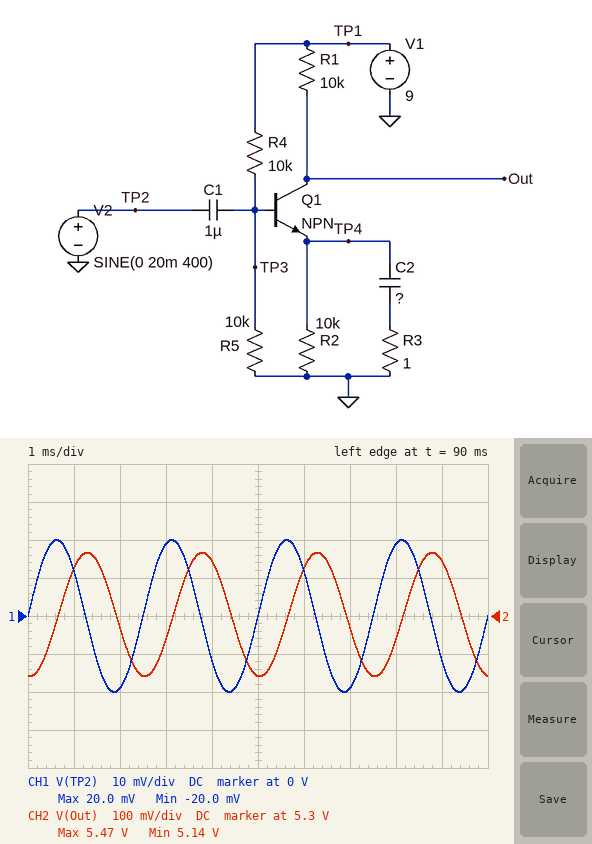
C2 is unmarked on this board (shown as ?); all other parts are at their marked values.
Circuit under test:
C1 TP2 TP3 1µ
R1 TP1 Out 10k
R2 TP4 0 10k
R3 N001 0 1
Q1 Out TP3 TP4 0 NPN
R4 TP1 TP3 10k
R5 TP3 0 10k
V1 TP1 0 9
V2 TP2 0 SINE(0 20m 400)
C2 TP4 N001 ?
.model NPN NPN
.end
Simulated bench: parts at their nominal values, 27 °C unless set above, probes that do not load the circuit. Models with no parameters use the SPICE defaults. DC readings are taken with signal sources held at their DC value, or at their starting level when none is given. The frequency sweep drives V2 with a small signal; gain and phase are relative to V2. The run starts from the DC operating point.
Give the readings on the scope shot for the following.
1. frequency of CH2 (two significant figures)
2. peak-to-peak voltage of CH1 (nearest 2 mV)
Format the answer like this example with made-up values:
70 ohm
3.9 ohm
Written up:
400 Hz
40 mV
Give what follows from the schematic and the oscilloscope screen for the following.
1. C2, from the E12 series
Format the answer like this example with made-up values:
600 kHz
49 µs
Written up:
330 nF
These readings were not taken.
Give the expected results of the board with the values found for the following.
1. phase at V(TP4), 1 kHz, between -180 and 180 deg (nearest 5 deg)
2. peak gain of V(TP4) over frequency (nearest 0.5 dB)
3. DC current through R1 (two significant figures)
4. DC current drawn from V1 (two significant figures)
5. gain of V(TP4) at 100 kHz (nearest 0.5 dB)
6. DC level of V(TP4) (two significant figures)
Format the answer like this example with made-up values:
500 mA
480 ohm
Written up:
-5 deg
0 dB
370 µA
820 µA
-23.0 dB
3.7 V
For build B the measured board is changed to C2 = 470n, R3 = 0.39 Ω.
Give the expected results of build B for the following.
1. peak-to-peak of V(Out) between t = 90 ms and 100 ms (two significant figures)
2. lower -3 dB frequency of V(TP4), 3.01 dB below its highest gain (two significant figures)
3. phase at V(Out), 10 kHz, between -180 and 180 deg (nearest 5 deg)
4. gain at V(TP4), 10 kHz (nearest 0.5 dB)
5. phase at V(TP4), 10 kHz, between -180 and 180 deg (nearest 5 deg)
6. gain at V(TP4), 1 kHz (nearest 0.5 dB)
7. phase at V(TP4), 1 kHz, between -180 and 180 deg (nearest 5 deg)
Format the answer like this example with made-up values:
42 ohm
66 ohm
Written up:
460 mV
31 Hz
-155 deg
-7.0 dB
-65 deg
-0.5 dB
-10 deg
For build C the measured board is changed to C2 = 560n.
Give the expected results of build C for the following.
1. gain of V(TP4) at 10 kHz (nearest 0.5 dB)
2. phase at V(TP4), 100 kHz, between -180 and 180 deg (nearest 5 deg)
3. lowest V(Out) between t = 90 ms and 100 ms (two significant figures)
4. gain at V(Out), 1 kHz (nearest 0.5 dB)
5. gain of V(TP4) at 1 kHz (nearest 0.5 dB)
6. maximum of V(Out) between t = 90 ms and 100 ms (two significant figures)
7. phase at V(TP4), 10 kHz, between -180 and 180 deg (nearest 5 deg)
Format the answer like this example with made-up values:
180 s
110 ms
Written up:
-8.5 dB
-70 deg
5.0 V
30.5 dB
-0.5 dB
5.6 V
-65 deg
